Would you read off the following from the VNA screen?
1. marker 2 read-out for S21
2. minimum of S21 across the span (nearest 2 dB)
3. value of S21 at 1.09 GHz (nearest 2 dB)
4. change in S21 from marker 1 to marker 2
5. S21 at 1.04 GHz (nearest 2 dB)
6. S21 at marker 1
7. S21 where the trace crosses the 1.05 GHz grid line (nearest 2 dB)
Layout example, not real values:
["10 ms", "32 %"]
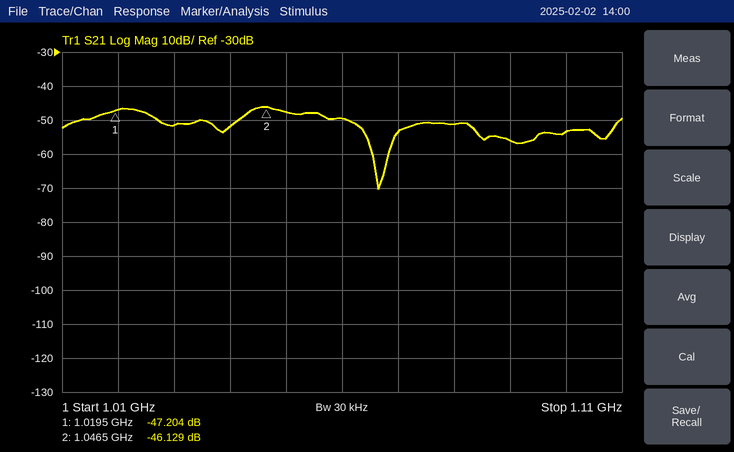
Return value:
["-46.129 dB", "-70 dB", "-56 dB", "1.075 dB", "-52 dB", "-47.204 dB", "-48 dB"]
